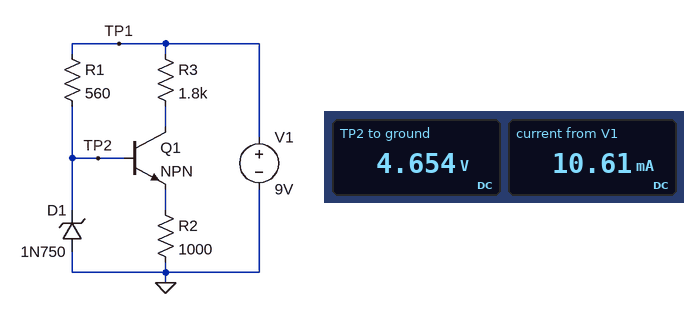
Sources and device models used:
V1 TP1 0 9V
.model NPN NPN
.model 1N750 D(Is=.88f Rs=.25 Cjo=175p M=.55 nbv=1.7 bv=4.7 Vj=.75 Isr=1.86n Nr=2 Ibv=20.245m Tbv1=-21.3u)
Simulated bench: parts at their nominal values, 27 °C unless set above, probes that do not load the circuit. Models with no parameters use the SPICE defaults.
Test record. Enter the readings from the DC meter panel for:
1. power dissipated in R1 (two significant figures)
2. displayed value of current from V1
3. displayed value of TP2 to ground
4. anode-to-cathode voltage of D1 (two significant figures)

34 mW
10.61 mA
4.654 V
-4.7 V
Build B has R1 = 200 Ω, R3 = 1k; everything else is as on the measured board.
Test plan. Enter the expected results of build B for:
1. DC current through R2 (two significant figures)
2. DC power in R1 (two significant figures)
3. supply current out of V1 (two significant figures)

3.9 mA
92 mW
25 mA
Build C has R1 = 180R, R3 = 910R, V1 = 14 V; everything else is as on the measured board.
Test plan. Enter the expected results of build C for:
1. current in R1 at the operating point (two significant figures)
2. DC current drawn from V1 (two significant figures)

51 mA
55 mA
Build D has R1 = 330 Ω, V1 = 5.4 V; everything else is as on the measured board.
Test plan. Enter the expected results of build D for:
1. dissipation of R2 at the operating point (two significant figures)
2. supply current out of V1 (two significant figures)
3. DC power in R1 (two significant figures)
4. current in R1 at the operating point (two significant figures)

13 mW
3.8 mA
2.6 mW
2.8 mA
